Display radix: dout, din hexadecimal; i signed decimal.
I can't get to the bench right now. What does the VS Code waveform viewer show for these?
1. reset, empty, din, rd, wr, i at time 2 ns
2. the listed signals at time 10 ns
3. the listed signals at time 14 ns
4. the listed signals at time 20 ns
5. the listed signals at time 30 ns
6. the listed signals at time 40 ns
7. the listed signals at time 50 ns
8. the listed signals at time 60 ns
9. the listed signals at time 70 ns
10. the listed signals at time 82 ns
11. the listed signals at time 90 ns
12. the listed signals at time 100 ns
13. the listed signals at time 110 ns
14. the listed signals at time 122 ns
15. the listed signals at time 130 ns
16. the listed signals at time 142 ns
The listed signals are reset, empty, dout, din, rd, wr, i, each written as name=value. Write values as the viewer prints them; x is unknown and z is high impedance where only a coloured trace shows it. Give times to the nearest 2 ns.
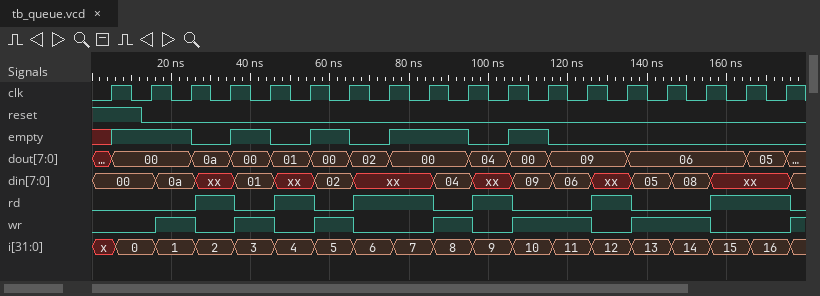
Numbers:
reset=1, empty=x, din=00, rd=0, wr=0, i=x
reset=1, empty=1, dout=00, din=00, rd=0, wr=0, i=0
reset=0, empty=1, dout=00, din=00, rd=0, wr=0, i=0
reset=0, empty=1, dout=00, din=0a, rd=0, wr=1, i=1
reset=0, empty=0, dout=0a, din=xx, rd=1, wr=0, i=2
reset=0, empty=1, dout=00, din=01, rd=0, wr=1, i=3
reset=0, empty=0, dout=01, din=xx, rd=1, wr=0, i=4
reset=0, empty=1, dout=00, din=02, rd=0, wr=1, i=5
reset=0, empty=0, dout=02, din=xx, rd=1, wr=0, i=6
reset=0, empty=1, dout=00, din=xx, rd=1, wr=0, i=7
reset=0, empty=1, dout=00, din=04, rd=0, wr=1, i=8
reset=0, empty=0, dout=04, din=xx, rd=1, wr=0, i=9
reset=0, empty=1, dout=00, din=09, rd=0, wr=1, i=10
reset=0, empty=0, dout=09, din=06, rd=0, wr=1, i=11
reset=0, empty=0, dout=09, din=xx, rd=1, wr=0, i=12
reset=0, empty=0, dout=06, din=05, rd=0, wr=1, i=13
